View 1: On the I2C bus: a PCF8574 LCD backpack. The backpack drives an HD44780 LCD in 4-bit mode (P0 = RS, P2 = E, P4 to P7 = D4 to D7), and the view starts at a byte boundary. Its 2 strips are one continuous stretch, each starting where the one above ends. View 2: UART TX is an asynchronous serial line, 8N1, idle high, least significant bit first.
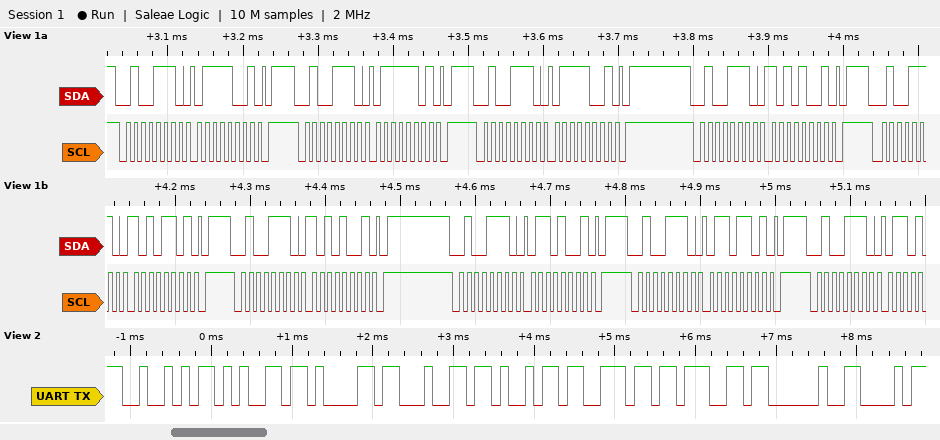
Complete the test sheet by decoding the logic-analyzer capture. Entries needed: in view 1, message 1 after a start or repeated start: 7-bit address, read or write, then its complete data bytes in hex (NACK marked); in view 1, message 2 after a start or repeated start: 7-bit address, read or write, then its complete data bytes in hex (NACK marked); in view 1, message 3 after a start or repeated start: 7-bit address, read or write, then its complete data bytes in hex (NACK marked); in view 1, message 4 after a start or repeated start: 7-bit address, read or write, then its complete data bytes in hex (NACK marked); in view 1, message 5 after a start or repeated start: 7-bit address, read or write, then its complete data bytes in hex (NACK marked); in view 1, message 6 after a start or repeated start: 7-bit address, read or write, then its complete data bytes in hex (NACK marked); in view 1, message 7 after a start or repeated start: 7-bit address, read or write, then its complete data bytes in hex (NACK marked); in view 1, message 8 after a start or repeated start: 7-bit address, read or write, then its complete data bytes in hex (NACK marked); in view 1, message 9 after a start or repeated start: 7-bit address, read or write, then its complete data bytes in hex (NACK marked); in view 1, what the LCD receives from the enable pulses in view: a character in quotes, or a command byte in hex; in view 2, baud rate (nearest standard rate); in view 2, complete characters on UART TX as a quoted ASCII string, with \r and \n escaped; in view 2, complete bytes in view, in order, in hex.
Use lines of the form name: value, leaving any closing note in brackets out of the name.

in view 1, message 1 after a start or repeated start: 7-bit address, read or write, then its complete data bytes in hex: 0x27 write: 79
in view 1, message 2 after a start or repeated start: 7-bit address, read or write, then its complete data bytes in hex: 0x27 write: 7D
in view 1, message 3 after a start or repeated start: 7-bit address, read or write, then its complete data bytes in hex: 0x27 write: 79
in view 1, message 4 after a start or repeated start: 7-bit address, read or write, then its complete data bytes in hex: 0x27 write: A9
in view 1, message 5 after a start or repeated start: 7-bit address, read or write, then its complete data bytes in hex: 0x27 write: AD
in view 1, message 6 after a start or repeated start: 7-bit address, read or write, then its complete data bytes in hex: 0x27 write: A9
in view 1, message 7 after a start or repeated start: 7-bit address, read or write, then its complete data bytes in hex: 0x27 write: 69
in view 1, message 8 after a start or repeated start: 7-bit address, read or write, then its complete data bytes in hex: 0x27 write: 6D
in view 1, message 9 after a start or repeated start: 7-bit address, read or write, then its complete data bytes in hex: 0x27 write
in view 1, what the LCD receives from the enable pulses in view: a character in quotes, or a command byte in hex: 'z'
in view 2, baud rate: 9600 baud
in view 2, complete characters on UART TX as a quoted ASCII string, with \r and \n escaped: "Reading "
in view 2, complete bytes in view, in order, in hex: 52 65 61 64 69 6E 67 20
